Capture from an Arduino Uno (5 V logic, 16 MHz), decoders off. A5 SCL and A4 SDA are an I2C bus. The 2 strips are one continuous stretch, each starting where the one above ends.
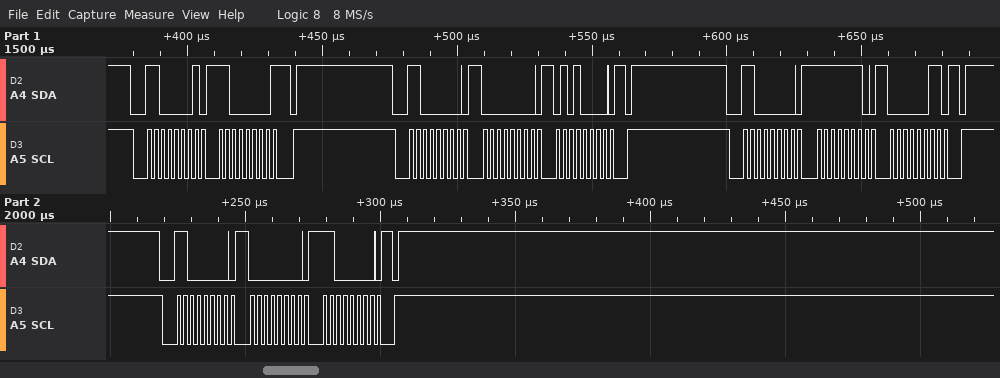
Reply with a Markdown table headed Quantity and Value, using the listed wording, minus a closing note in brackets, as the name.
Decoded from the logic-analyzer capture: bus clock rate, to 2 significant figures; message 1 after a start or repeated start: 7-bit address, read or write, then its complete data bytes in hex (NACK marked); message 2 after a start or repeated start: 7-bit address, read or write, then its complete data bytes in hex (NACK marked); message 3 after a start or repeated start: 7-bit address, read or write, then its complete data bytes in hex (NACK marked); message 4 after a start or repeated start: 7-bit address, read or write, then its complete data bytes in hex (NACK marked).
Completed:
| Quantity | Value |
|---|---|
| bus clock rate, to 2 significant figures | 400 kHz |
| message 1 after a start or repeated start: 7-bit address, read or write, then its complete data bytes in hex | 0x60 read: C0 NACK |
| message 2 after a start or repeated start: 7-bit address, read or write, then its complete data bytes in hex | 0x60 write: 00 50 |
| message 3 after a start or repeated start: 7-bit address, read or write, then its complete data bytes in hex | 0x60 write: FE 03 |
| message 4 after a start or repeated start: 7-bit address, read or write, then its complete data bytes in hex | 0x60 write: 00 C0 |
